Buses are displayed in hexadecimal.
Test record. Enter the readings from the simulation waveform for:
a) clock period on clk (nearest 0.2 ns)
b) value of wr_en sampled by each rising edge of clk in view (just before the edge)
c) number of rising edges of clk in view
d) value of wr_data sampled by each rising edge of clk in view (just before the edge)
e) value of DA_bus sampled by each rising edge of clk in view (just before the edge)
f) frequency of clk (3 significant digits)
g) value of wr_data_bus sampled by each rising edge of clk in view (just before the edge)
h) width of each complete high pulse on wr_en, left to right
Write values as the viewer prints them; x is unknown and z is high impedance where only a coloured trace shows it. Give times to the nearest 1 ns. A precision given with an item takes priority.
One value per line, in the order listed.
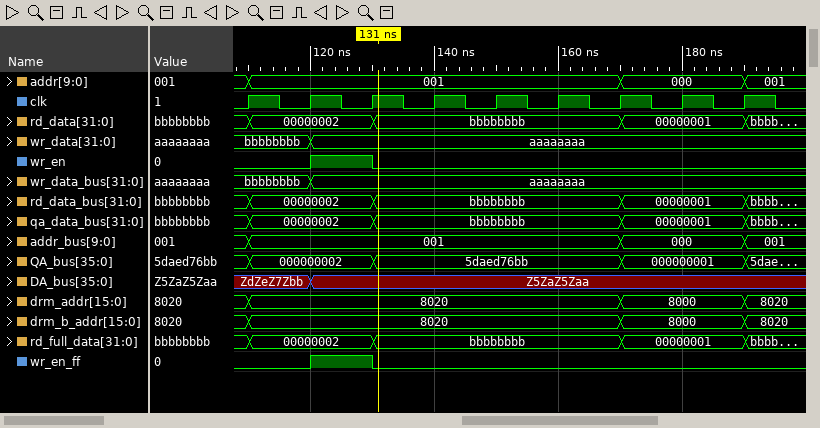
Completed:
10 ns
0 0 1 0 0 0 0 0 0
9
bbbbbbbb, bbbbbbbb, aaaaaaaa, aaaaaaaa, aaaaaaaa, aaaaaaaa, aaaaaaaa, aaaaaaaa, aaaaaaaa
ZdZeZ7Zbb, ZdZeZ7Zbb, Z5ZaZ5Zaa, Z5ZaZ5Zaa, Z5ZaZ5Zaa, Z5ZaZ5Zaa, Z5ZaZ5Zaa, Z5ZaZ5Zaa, Z5ZaZ5Zaa
100 MHz
bbbbbbbb, bbbbbbbb, aaaaaaaa, aaaaaaaa, aaaaaaaa, aaaaaaaa, aaaaaaaa, aaaaaaaa, aaaaaaaa
10 ns
